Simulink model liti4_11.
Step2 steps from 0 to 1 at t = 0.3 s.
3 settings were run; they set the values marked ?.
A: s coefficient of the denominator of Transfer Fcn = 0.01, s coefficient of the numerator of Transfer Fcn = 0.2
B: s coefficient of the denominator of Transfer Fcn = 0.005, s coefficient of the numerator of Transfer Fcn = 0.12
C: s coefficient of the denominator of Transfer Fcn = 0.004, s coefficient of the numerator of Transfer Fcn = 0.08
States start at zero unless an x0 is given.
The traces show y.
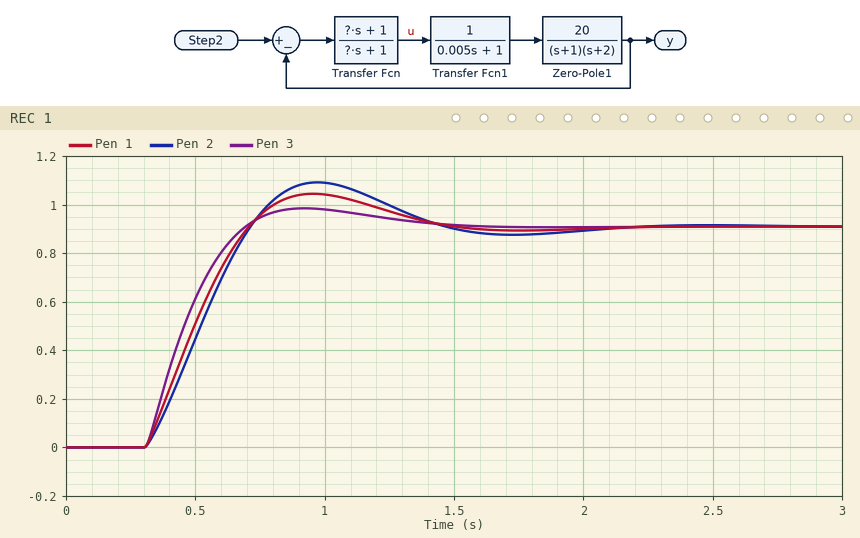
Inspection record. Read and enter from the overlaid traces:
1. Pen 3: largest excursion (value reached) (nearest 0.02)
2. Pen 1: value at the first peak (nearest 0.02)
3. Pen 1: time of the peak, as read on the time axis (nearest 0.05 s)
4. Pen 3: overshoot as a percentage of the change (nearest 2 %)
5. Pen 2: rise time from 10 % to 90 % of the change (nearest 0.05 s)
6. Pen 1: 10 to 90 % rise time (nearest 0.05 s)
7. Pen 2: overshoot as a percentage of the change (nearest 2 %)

0.98
1.04
0.95 s
8 %
0.30 s
0.30 s
20 %
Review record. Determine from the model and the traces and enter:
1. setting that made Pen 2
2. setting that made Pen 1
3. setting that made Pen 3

C
B
A
